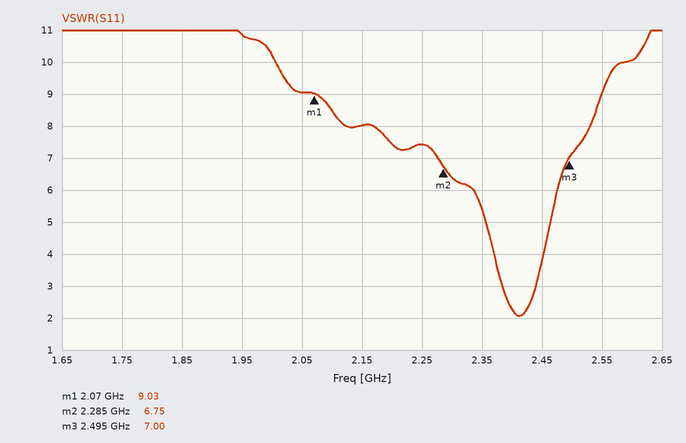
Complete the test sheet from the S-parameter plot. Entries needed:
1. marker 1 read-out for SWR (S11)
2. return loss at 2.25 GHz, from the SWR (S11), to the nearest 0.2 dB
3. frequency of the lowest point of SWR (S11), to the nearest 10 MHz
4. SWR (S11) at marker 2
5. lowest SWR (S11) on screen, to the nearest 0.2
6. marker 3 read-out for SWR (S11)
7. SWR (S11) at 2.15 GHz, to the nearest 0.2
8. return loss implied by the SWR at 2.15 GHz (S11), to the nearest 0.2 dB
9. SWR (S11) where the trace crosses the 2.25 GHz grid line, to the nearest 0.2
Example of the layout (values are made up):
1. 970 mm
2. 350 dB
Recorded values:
1. 9.03
2. 2.4 dB
3. 2.41 GHz
4. 6.75
5. 2.0
6. 7.00
7. 8.0
8. 2.2 dB
9. 7.4
